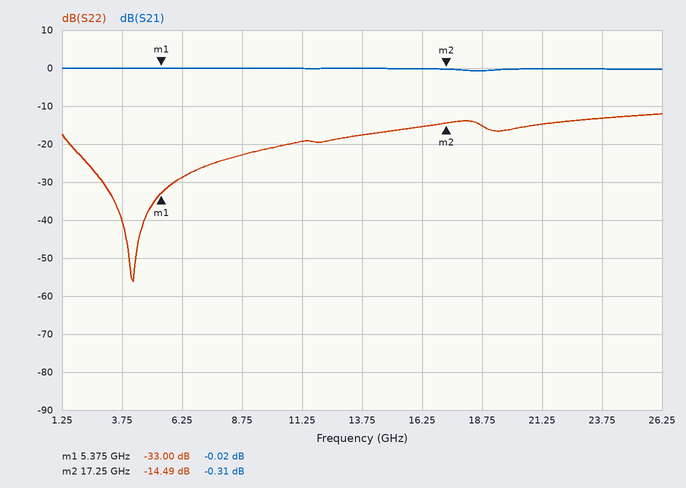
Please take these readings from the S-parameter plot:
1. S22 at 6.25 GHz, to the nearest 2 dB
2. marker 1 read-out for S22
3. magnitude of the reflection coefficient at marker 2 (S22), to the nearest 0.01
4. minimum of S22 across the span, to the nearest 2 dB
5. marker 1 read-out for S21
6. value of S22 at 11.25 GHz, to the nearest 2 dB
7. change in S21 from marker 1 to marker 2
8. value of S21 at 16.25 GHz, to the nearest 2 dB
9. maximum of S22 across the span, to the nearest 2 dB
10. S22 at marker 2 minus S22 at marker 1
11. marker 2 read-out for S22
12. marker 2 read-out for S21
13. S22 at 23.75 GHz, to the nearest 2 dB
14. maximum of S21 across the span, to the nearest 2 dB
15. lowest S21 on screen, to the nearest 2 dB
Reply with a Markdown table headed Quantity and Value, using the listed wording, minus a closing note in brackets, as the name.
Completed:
| Quantity | Value |
|---|---|
| S22 at 6.25 GHz, to the nearest 2 dB | -28 dB |
| marker 1 read-out for S22 | -33.00 dB |
| magnitude of the reflection coefficient at marker 2 (S22), to the nearest 0.01 | 0.19 |
| minimum of S22 across the span, to the nearest 2 dB | -56 dB |
| marker 1 read-out for S21 | -0.02 dB |
| value of S22 at 11.25 GHz, to the nearest 2 dB | -20 dB |
| change in S21 from marker 1 to marker 2 | -0.29 dB |
| value of S21 at 16.25 GHz, to the nearest 2 dB | 0 dB |
| maximum of S22 across the span, to the nearest 2 dB | -12 dB |
| S22 at marker 2 minus S22 at marker 1 | 18.51 dB |
| marker 2 read-out for S22 | -14.49 dB |
| marker 2 read-out for S21 | -0.31 dB |
| S22 at 23.75 GHz, to the nearest 2 dB | -14 dB |
| maximum of S21 across the span, to the nearest 2 dB | 0 dB |
| lowest S21 on screen, to the nearest 2 dB | 0 dB |
